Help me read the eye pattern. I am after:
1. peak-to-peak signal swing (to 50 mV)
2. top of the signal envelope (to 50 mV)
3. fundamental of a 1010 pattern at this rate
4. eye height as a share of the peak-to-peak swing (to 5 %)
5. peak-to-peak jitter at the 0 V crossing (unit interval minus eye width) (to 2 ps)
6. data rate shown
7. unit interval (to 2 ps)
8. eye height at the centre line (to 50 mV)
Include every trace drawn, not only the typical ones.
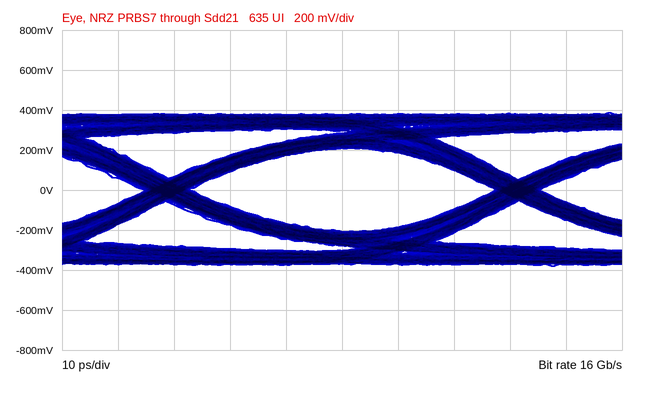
750 mV
400 mV
8 GHz
55 %
8 ps
16 Gb/s
62 ps
400 mV
